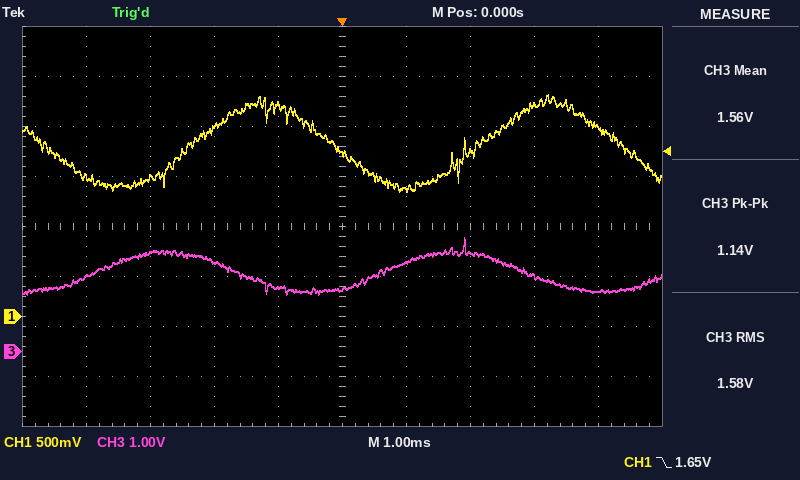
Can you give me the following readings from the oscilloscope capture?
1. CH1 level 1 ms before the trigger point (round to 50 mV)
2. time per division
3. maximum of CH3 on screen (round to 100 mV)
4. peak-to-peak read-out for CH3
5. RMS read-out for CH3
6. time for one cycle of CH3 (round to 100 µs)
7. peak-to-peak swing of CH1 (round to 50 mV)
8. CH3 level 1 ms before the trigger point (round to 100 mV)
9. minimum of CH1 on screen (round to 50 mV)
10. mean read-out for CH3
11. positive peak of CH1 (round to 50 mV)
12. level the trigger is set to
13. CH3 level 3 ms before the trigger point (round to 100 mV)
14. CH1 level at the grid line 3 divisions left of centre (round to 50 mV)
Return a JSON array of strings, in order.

["2.10 V", "1 ms", "2.3 V", "1.14 V", "1.58 V", "4.5 ms", "950 mV", "1.3 V", "1.25 V", "1.56 V", "2.20 V", "1.65 V", "2.0 V", "1.40 V"]
